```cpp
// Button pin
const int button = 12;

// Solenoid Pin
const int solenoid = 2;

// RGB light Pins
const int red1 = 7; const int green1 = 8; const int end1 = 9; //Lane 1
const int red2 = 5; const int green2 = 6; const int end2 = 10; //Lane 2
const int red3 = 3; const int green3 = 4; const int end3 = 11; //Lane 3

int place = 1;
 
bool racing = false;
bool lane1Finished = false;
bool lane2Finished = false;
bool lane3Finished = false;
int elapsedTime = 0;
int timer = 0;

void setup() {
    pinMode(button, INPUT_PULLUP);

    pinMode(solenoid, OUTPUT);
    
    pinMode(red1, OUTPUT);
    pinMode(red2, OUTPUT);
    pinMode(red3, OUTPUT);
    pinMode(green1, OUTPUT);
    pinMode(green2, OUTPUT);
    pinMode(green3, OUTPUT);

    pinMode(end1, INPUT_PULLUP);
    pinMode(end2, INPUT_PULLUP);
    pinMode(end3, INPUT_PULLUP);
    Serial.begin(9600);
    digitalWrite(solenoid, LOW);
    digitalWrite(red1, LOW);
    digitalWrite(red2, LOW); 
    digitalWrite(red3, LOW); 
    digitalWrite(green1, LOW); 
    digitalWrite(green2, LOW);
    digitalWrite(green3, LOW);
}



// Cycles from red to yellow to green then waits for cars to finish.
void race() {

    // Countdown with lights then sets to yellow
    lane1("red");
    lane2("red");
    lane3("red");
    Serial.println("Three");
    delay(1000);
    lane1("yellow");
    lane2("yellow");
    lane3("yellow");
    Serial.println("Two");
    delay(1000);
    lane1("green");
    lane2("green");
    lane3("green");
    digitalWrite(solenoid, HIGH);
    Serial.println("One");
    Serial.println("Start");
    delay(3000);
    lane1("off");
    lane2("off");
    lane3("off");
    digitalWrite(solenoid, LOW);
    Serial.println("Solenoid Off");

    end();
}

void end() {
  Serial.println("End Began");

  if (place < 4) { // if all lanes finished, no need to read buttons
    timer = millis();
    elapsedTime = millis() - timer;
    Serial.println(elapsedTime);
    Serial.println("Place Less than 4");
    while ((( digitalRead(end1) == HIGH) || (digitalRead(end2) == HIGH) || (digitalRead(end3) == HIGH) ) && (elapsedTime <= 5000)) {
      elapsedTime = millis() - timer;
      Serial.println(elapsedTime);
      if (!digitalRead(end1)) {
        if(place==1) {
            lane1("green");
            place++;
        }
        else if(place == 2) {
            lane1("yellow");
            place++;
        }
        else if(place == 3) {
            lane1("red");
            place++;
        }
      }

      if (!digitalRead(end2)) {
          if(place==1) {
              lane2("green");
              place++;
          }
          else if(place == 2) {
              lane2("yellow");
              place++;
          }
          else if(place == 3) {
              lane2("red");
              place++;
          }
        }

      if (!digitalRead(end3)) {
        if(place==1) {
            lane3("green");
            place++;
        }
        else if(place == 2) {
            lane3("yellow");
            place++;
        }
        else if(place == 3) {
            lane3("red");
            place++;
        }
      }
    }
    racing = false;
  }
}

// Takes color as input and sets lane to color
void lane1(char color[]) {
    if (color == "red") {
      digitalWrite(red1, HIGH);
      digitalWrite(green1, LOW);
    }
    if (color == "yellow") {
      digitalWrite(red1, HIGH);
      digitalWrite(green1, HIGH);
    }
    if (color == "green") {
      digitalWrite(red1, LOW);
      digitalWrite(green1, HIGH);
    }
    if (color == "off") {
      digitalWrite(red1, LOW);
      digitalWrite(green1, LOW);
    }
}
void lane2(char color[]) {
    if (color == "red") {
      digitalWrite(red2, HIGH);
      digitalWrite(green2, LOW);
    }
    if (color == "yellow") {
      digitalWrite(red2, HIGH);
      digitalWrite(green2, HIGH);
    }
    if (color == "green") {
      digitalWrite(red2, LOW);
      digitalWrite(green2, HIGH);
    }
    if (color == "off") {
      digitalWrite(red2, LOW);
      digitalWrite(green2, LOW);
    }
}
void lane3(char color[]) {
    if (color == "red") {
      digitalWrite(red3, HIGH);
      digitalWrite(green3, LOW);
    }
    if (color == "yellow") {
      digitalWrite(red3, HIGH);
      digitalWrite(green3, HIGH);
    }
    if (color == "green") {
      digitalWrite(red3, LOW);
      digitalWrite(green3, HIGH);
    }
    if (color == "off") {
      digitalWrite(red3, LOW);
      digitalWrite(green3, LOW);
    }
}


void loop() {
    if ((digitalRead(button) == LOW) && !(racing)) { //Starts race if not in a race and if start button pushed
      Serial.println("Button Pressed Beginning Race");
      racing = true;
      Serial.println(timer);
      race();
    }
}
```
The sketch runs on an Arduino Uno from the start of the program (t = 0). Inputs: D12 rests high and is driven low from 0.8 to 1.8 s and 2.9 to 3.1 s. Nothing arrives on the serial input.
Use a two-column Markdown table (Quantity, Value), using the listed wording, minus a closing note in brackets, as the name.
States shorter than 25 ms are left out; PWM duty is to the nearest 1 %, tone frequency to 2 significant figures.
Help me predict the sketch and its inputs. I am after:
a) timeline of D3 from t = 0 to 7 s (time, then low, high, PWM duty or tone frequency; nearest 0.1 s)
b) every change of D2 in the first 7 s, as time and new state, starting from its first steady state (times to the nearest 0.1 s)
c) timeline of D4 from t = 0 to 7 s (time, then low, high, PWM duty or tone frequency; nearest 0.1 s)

| Quantity | Value |
|---|---|
| timeline of D3 from t = 0 to 7 s | 0 s low; 0.8 s high; 2.8 s low |
| every change of D2 in the first 7 s, as time and new state, starting from its first steady state | 0 s low; 2.8 s high; 5.8 s low |
| timeline of D4 from t = 0 to 7 s | 0 s low; 1.8 s high; 5.8 s low |
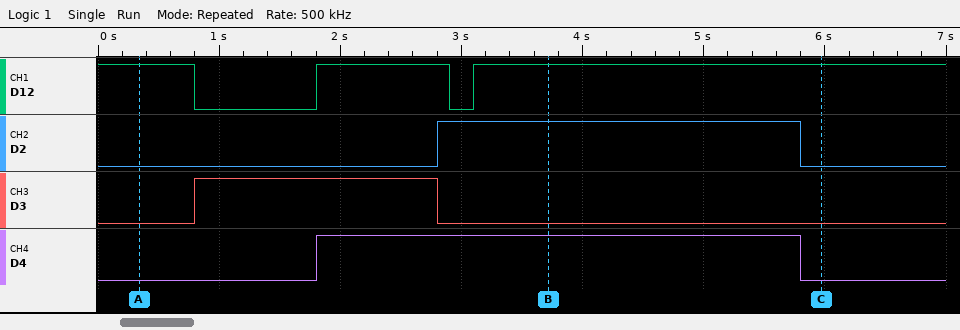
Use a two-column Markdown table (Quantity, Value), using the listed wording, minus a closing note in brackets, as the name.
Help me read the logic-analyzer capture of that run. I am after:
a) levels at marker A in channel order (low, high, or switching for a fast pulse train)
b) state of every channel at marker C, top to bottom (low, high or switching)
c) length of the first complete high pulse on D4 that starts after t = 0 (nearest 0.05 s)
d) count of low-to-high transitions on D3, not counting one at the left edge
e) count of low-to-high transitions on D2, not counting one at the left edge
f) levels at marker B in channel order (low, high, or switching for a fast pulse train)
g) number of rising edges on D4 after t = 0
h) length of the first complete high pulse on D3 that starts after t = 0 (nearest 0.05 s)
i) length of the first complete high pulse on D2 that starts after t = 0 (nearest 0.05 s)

| Quantity | Value |
|---|---|
| levels at marker A in channel order | D12 high, D2 low, D3 low, D4 low |
| state of every channel at marker C, top to bottom | D12 high, D2 low, D3 low, D4 low |
| length of the first complete high pulse on D4 that starts after t = 0 | 4.00 s |
| count of low-to-high transitions on D3, not counting one at the left edge | 1 |
| count of low-to-high transitions on D2, not counting one at the left edge | 1 |
| levels at marker B in channel order | D12 high, D2 high, D3 low, D4 high |
| number of rising edges on D4 after t = 0 | 1 |
| length of the first complete high pulse on D3 that starts after t = 0 | 2.00 s |
| length of the first complete high pulse on D2 that starts after t = 0 | 3.00 s |
